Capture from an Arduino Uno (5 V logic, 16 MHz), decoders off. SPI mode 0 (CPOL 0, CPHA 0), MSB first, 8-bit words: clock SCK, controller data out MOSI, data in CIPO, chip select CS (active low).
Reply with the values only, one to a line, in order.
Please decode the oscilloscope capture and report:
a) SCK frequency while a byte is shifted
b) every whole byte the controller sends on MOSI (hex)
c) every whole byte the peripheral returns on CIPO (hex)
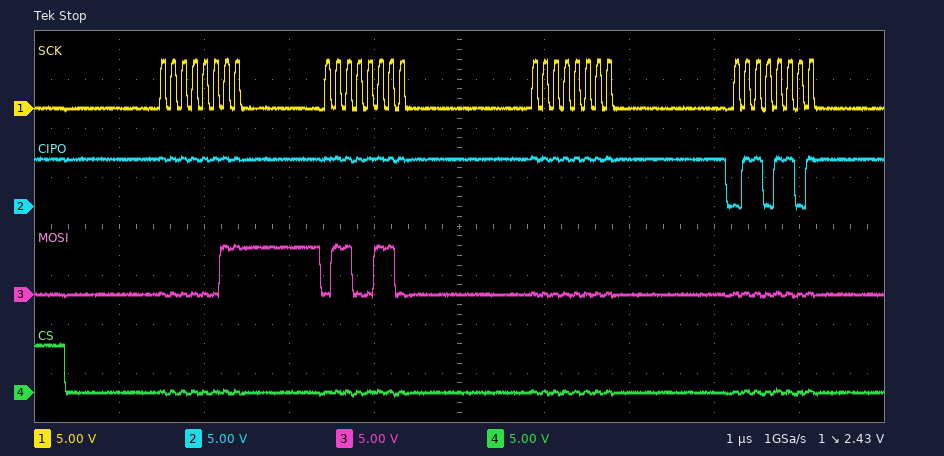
8 MHz
03 66 00 00
FF FF FF 6D
